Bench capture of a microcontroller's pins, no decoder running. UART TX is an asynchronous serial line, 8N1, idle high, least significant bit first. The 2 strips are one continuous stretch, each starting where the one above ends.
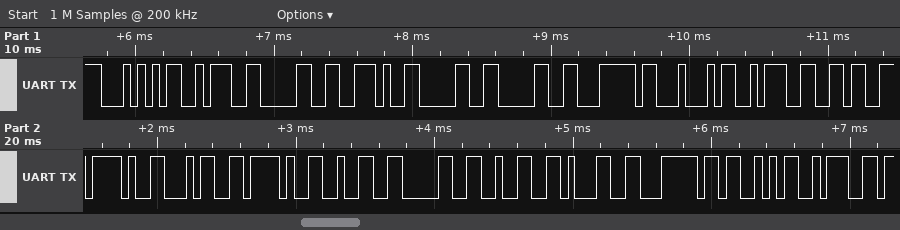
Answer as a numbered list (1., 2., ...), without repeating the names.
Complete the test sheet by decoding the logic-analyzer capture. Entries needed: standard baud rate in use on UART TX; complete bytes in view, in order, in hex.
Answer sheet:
1. 19200 baud
2. 54 3A 30 2E 30 30 7C 44 3A 36 2F 34 2F 32 30 32 31 7C 53 3A
